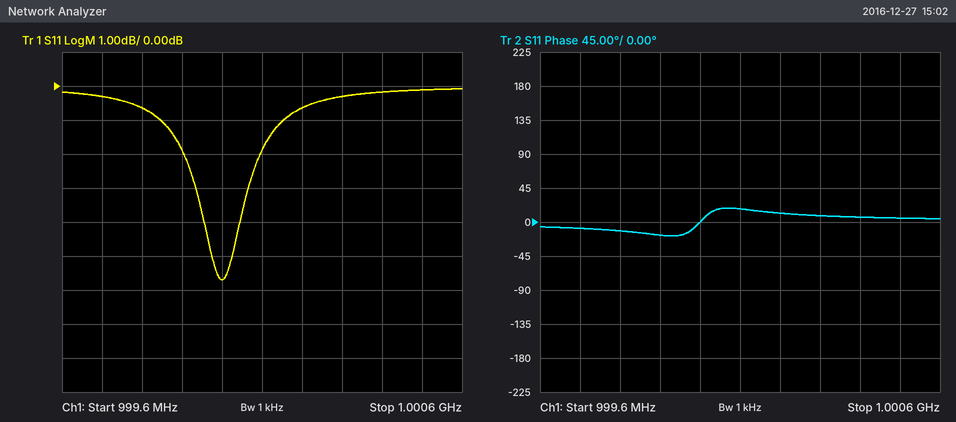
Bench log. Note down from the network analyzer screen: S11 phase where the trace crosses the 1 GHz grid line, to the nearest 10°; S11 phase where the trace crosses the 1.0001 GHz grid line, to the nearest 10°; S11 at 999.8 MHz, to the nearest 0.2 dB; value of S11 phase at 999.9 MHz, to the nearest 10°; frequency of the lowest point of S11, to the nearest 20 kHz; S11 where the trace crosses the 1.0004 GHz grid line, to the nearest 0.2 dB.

0°
20°
-0.6 dB
-20°
1.00000 GHz
-0.2 dB
